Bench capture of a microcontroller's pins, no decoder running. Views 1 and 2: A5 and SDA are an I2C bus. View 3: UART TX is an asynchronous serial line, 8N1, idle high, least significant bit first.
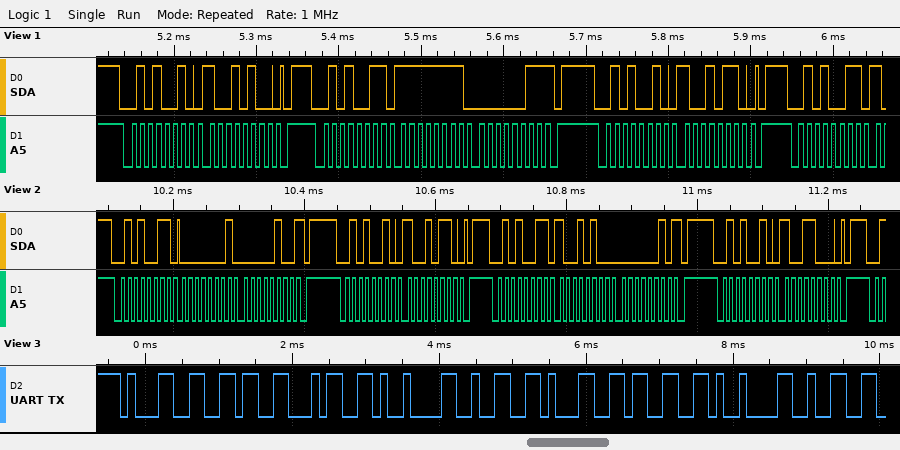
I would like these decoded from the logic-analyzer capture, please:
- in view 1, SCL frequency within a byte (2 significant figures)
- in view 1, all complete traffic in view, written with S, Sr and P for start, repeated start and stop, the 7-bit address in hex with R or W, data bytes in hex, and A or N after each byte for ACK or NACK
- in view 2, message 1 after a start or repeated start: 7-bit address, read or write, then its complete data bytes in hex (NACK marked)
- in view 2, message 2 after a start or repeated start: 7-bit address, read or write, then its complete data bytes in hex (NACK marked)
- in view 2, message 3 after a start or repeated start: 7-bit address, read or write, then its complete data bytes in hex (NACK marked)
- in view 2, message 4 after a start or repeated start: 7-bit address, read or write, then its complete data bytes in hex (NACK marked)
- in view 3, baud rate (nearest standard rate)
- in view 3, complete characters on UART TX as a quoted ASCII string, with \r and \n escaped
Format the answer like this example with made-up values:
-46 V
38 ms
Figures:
100 kHz
S 29W A 94 A P S 29R A FF A 03 N P S 29W A 96 A P S 29R A
0x29 read: 01 04 NACK
0x29 write: 96
0x29 read: 94 02 NACK
0x29 write: 98
9600 baud
"164\t213\t2"
